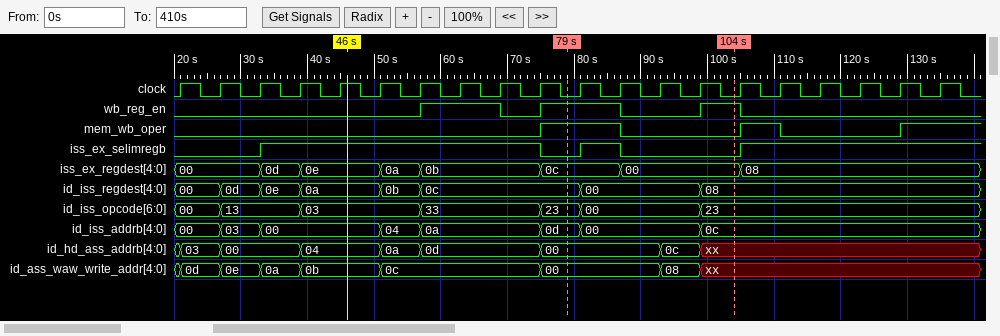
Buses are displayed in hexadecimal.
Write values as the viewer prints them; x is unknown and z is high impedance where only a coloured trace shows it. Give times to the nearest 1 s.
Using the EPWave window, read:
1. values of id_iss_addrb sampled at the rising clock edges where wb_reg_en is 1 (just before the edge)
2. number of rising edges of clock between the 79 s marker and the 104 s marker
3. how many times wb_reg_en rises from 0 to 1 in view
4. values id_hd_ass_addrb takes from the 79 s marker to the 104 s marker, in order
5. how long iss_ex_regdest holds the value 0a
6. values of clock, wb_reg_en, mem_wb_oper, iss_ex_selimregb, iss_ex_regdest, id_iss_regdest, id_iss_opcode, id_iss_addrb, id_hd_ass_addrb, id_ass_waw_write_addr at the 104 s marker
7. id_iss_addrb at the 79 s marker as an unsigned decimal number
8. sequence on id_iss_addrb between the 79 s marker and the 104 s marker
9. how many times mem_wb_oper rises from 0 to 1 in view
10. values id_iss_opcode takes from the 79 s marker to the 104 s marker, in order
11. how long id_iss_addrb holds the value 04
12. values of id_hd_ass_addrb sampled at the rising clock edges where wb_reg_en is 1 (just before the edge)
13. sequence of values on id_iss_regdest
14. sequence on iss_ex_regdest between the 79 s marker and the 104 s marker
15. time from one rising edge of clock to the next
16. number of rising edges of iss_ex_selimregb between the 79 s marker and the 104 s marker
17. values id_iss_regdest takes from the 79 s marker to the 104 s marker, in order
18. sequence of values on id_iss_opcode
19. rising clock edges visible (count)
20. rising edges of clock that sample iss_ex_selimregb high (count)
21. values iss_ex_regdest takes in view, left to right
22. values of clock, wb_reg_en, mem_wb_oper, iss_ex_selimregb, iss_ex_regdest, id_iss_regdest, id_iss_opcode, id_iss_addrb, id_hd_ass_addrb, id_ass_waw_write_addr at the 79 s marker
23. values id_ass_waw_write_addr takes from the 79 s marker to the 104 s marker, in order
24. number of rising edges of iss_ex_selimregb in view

0a, 0a, 0d, 00, 0c
4
3
00, 0c, xx
6 s
clock=0, wb_reg_en=1, mem_wb_oper=0, iss_ex_selimregb=0, iss_ex_regdest=00, id_iss_regdest=08, id_iss_opcode=23, id_iss_addrb=0c, id_hd_ass_addrb=xx, id_ass_waw_write_addr=xx
13
0d, 00, 0c
3
23, 00, 23
6 s
0d, 0d, 00, 00, xx
00, 0d, 0e, 0a, 0b, 0c, 00, 08
0c, 00
6 s
1
0c, 00, 08
00, 13, 03, 33, 23, 00, 23
20
13
00, 0d, 0e, 0a, 0b, 0c, 00, 08
clock=0, wb_reg_en=1, mem_wb_oper=1, iss_ex_selimregb=0, iss_ex_regdest=0c, id_iss_regdest=0c, id_iss_opcode=23, id_iss_addrb=0d, id_hd_ass_addrb=00, id_ass_waw_write_addr=00
00, 08, xx
3
